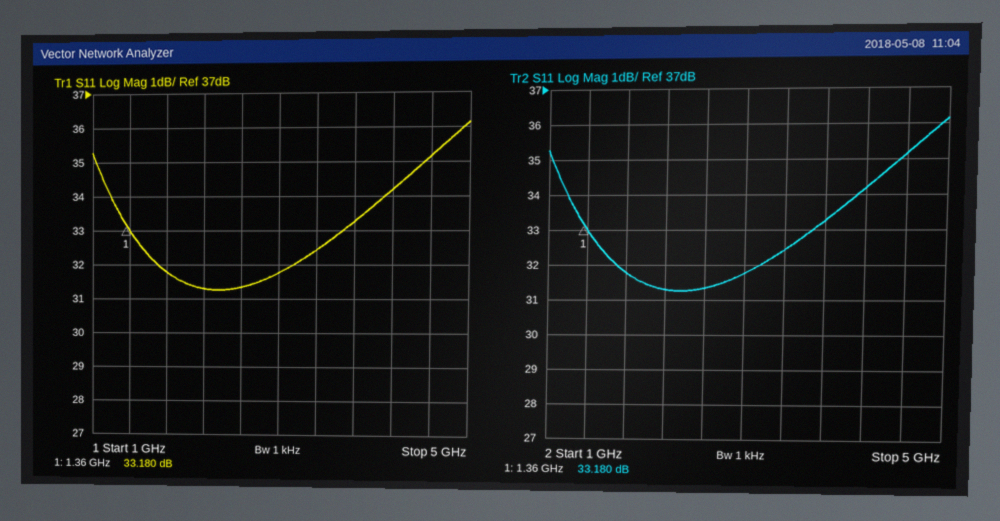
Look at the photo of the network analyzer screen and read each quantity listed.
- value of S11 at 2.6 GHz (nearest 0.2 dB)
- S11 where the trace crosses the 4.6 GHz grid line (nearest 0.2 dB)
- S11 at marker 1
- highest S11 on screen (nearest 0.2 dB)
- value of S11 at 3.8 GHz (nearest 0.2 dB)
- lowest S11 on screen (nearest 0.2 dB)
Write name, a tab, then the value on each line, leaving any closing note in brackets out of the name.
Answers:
value of S11 at 2.6 GHz	31.4 dB
S11 where the trace crosses the 4.6 GHz grid line	35.2 dB
S11 at marker 1	33.180 dB
highest S11 on screen	36.2 dB
value of S11 at 3.8 GHz	33.2 dB
lowest S11 on screen	31.2 dB
